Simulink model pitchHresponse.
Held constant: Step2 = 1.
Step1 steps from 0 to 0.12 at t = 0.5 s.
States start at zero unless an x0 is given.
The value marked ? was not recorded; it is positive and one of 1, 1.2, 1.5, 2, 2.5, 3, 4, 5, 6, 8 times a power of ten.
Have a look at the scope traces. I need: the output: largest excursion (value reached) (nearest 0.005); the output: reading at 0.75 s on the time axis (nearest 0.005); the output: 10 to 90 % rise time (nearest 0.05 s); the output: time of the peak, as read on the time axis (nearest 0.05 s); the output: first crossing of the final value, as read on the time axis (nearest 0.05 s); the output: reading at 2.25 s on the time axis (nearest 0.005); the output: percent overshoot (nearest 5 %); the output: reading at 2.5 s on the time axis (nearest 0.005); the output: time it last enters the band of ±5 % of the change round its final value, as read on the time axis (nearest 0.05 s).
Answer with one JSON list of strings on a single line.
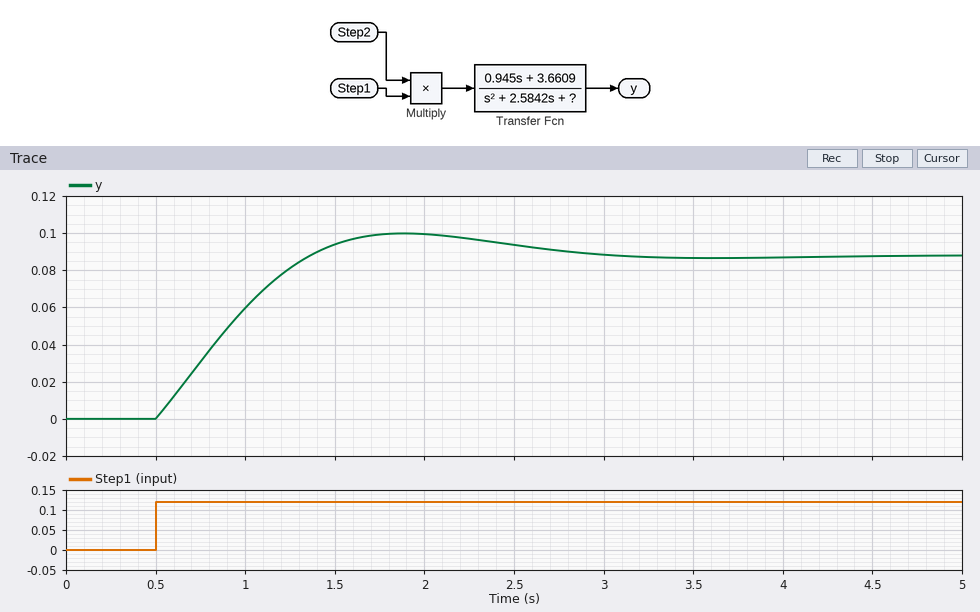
["0.100", "0.030", "0.65 s", "1.90 s", "1.35 s", "0.095", "15 %", "0.095", "2.60 s"]
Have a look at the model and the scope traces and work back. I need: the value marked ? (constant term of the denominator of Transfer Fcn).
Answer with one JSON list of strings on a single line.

["5"]
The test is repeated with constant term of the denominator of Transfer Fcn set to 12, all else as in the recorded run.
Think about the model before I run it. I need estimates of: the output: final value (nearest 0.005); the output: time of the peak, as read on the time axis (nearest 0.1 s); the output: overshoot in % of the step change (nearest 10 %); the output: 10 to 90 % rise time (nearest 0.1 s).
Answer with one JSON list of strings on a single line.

["0.035", "1.2 s", "40 %", "0.3 s"]
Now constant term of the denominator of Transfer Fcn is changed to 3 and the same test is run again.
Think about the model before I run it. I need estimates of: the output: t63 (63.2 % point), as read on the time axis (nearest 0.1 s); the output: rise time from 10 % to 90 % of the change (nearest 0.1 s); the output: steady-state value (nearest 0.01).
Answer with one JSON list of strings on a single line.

["1.3 s", "1.2 s", "0.15"]
